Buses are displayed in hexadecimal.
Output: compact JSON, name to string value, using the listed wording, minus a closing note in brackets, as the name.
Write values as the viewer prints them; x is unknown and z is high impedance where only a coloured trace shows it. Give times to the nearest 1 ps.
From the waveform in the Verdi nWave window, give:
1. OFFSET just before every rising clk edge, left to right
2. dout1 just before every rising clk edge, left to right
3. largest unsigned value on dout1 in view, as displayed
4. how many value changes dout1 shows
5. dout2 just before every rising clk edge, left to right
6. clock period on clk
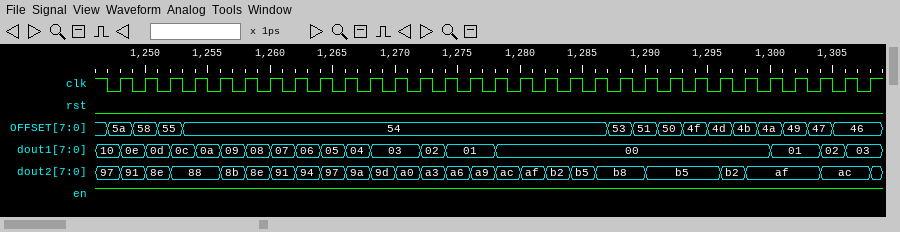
{"OFFSET just before every rising clk edge, left to right": "5a, 58, 55, 54, 54, 54, 54, 54, 54, 54, 54, 54, 54, 54, 54, 54, 54, 54, 54, 54, 53, 51, 50, 4f, 4d, 4b, 4a, 49, 47, 46, 46", "dout1 just before every rising clk edge, left to right": "10, 0e, 0d, 0c, 0a, 09, 08, 07, 06, 05, 04, 03, 03, 02, 01, 01, 00, 00, 00, 00, 00, 00, 00, 00, 00, 00, 00, 01, 01, 02, 03", "largest unsigned value on dout1 in view, as displayed": "10", "how many value changes dout1 shows": "17", "dout2 just before every rising clk edge, left to right": "97, 91, 8e, 88, 88, 8b, 8e, 91, 94, 97, 9a, 9d, a0, a3, a6, a9, ac, af, b2, b5, b8, b8, b5, b5, b5, b2, af, af, af, ac, ac", "clock period on clk": "2 ps"}
